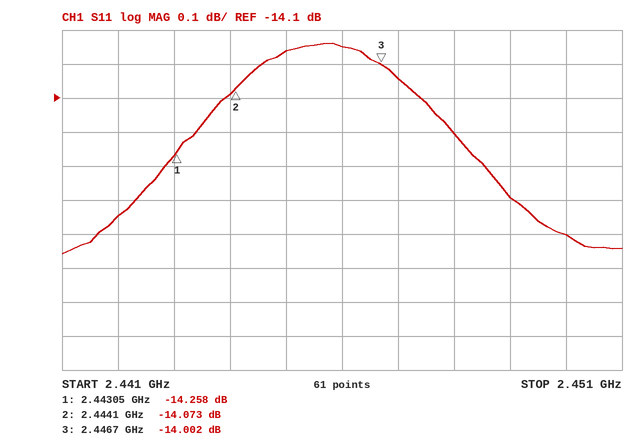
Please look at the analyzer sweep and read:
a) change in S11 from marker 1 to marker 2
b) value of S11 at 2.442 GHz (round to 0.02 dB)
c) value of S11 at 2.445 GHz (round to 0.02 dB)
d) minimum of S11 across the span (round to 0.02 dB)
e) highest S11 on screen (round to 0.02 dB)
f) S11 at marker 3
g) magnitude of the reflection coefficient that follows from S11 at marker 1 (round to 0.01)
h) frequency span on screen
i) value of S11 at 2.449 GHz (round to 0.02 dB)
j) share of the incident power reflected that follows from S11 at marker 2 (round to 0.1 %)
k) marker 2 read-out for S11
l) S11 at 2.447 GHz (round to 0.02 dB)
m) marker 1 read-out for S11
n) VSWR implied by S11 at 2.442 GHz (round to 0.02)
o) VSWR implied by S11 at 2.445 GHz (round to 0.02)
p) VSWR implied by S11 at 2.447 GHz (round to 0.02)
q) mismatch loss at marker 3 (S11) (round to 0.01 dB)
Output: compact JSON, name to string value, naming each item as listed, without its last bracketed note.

{"change in S11 from marker 1 to marker 2": "0.185 dB", "value of S11 at 2.442 GHz": "-14.44 dB", "value of S11 at 2.445 GHz": "-13.96 dB", "minimum of S11 across the span": "-14.56 dB", "highest S11 on screen": "-13.94 dB", "S11 at marker 3": "-14.002 dB", "magnitude of the reflection coefficient that follows from S11 at marker 1": "0.19", "frequency span on screen": "10 MHz", "value of S11 at 2.449 GHz": "-14.40 dB", "share of the incident power reflected that follows from S11 at marker 2": "3.9 %", "marker 2 read-out for S11": "-14.073 dB", "S11 at 2.447 GHz": "-14.04 dB", "marker 1 read-out for S11": "-14.258 dB", "VSWR implied by S11 at 2.442 GHz": "1.46", "VSWR implied by S11 at 2.445 GHz": "1.50", "VSWR implied by S11 at 2.447 GHz": "1.50", "mismatch loss at marker 3 (S11)": "0.18 dB"}
